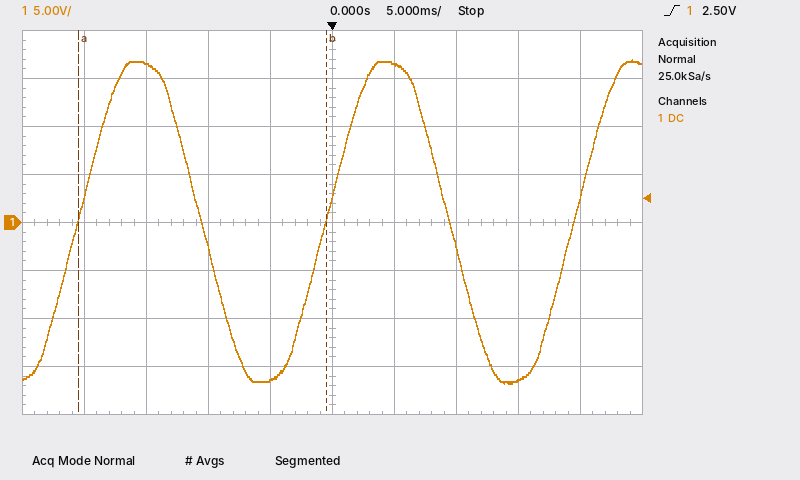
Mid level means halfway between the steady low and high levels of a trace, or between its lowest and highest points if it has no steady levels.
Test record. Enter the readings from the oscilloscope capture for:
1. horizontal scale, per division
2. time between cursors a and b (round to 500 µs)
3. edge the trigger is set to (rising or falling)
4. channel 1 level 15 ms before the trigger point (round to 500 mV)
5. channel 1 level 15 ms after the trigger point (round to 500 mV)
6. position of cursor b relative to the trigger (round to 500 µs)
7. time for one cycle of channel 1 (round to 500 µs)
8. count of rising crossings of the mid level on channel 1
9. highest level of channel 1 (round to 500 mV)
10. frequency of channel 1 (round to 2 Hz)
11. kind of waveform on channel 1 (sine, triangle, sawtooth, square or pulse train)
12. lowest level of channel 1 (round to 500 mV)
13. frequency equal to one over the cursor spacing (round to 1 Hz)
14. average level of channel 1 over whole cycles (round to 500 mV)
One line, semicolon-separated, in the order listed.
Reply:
5 ms; 20.0 ms; rising; 16.5 V; -16.5 V; -500 µs; 20.0 ms; 3; 17.0 V; 50 Hz; sine; -17.0 V; 50 Hz; 0.0 V
